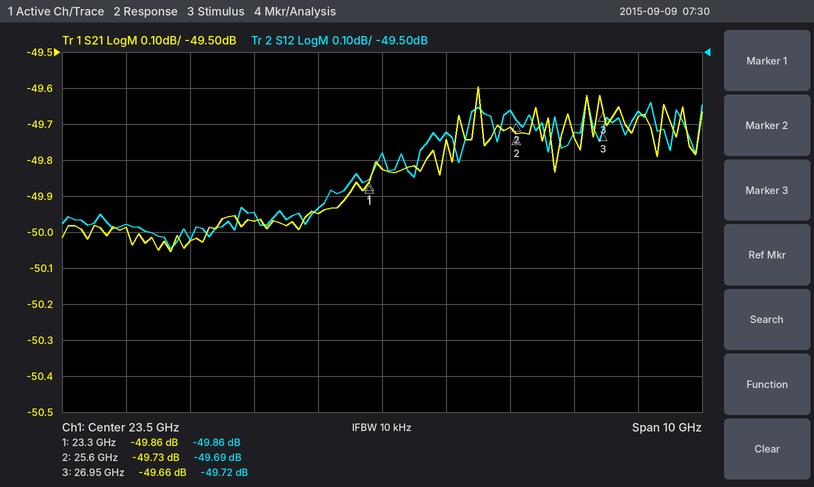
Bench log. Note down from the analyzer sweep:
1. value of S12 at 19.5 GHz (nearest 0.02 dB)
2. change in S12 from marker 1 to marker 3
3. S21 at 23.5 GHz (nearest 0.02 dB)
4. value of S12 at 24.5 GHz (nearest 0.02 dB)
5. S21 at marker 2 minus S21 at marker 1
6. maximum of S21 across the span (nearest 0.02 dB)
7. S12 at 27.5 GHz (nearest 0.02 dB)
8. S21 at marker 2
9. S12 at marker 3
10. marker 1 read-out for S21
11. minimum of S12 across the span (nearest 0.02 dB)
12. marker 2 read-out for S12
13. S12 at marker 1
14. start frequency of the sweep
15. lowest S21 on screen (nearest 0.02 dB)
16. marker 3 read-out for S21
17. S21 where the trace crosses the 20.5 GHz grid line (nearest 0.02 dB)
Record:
-49.98 dB
0.14 dB
-49.82 dB
-49.72 dB
0.13 dB
-49.60 dB
-49.66 dB
-49.73 dB
-49.72 dB
-49.86 dB
-50.04 dB
-49.69 dB
-49.86 dB
18.5 GHz
-50.06 dB
-49.66 dB
-50.02 dB
